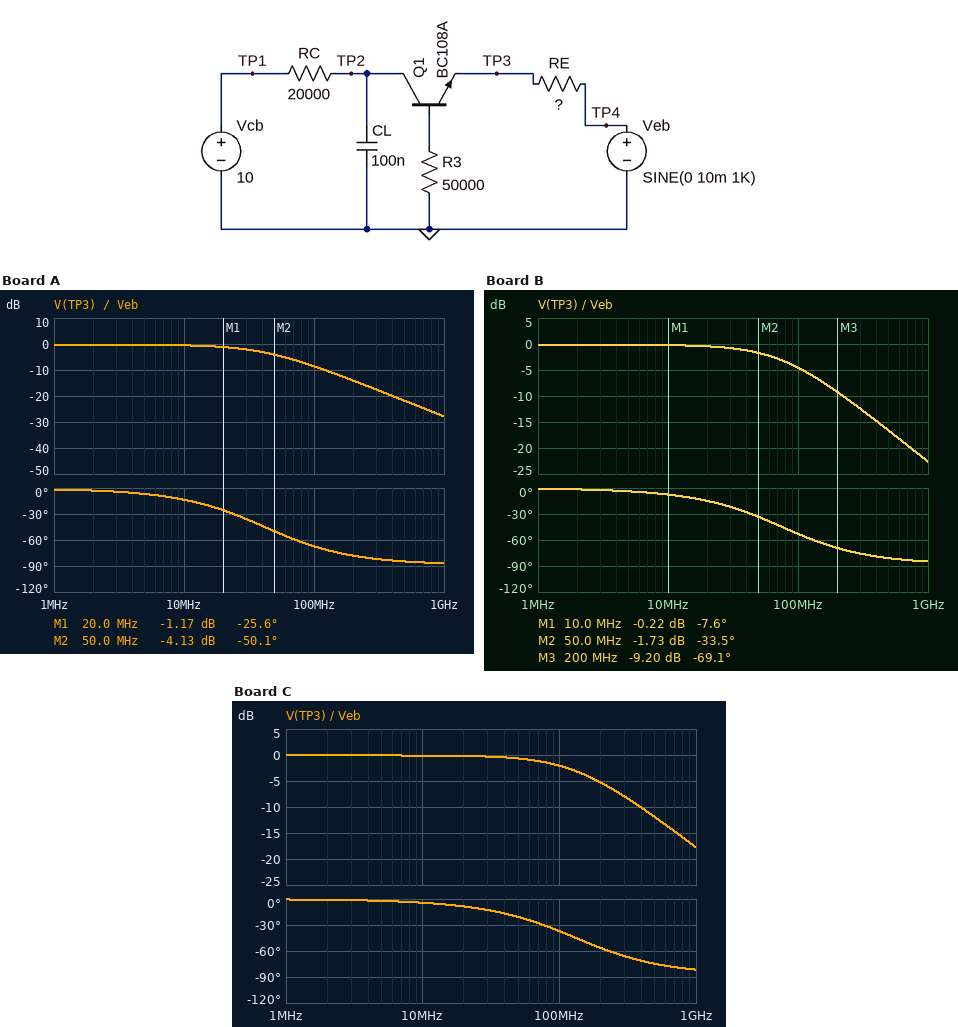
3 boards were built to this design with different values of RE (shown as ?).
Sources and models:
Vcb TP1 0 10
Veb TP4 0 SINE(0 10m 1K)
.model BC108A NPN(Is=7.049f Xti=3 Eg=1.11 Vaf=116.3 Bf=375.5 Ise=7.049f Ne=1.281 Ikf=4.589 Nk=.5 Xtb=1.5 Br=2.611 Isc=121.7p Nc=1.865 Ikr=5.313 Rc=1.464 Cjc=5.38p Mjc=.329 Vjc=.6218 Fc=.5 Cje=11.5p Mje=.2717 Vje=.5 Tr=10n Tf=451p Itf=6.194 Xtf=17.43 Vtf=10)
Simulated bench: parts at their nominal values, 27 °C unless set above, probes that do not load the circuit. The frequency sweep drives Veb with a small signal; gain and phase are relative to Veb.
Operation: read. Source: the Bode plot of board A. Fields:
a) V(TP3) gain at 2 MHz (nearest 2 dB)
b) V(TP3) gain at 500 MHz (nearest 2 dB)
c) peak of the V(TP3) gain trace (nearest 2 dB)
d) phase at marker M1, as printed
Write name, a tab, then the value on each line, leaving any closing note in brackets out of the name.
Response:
V(TP3) gain at 2 MHz	0 dB
V(TP3) gain at 500 MHz	-22 dB
peak of the V(TP3) gain trace	0 dB
phase at marker M1, as printed	-25.6 deg
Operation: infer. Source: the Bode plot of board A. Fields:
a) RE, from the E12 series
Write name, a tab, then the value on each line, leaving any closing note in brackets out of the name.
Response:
RE, from the E12 series	2.2 kΩ
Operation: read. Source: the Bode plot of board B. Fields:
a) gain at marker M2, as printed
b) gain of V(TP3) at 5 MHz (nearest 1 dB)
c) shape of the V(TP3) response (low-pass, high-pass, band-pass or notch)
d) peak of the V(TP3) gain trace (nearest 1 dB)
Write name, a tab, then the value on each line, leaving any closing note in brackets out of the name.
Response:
gain at marker M2, as printed	-1.73 dB
gain of V(TP3) at 5 MHz	0 dB
shape of the V(TP3) response	low-pass
peak of the V(TP3) gain trace	0 dB
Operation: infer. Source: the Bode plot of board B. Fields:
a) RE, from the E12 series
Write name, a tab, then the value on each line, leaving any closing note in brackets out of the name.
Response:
RE, from the E12 series	1.2 kΩ
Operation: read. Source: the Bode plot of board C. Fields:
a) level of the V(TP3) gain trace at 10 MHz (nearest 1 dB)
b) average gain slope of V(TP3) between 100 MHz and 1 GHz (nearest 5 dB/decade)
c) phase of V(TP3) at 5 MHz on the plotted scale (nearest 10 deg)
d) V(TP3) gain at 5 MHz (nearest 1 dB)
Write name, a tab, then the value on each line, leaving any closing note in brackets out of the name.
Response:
level of the V(TP3) gain trace at 10 MHz	0 dB
average gain slope of V(TP3) between 100 MHz and 1 GHz	-15 dB/decade
phase of V(TP3) at 5 MHz on the plotted scale	0 deg
V(TP3) gain at 5 MHz	0 dB
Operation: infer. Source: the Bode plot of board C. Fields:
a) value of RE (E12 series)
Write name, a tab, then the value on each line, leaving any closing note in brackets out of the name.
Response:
value of RE	680 Ω
